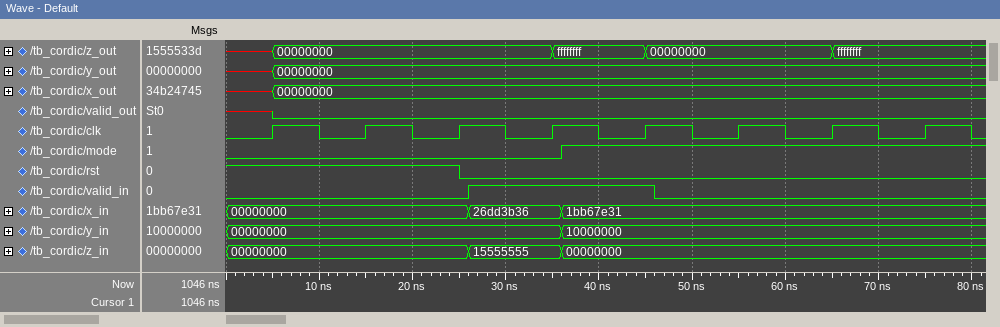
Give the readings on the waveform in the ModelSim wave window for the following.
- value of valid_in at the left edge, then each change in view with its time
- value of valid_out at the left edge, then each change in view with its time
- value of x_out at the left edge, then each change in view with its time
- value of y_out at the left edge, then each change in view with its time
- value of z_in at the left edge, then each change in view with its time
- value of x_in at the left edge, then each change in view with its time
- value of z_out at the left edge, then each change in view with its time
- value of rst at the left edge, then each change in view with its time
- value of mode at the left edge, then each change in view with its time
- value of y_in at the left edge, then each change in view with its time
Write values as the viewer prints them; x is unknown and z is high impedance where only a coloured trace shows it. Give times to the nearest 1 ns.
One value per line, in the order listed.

0, 1 at 26 ns, 0 at 46 ns
x, 0 at 5 ns
x, 00000000 at 5 ns
x, 00000000 at 5 ns
00000000, 15555555 at 26 ns, 00000000 at 36 ns
00000000, 26dd3b36 at 26 ns, 1bb67e31 at 36 ns
x, 00000000 at 5 ns, ffffffff at 35 ns, 00000000 at 45 ns, ffffffff at 65 ns
1, 0 at 25 ns
0, 1 at 36 ns
00000000, 10000000 at 36 ns
